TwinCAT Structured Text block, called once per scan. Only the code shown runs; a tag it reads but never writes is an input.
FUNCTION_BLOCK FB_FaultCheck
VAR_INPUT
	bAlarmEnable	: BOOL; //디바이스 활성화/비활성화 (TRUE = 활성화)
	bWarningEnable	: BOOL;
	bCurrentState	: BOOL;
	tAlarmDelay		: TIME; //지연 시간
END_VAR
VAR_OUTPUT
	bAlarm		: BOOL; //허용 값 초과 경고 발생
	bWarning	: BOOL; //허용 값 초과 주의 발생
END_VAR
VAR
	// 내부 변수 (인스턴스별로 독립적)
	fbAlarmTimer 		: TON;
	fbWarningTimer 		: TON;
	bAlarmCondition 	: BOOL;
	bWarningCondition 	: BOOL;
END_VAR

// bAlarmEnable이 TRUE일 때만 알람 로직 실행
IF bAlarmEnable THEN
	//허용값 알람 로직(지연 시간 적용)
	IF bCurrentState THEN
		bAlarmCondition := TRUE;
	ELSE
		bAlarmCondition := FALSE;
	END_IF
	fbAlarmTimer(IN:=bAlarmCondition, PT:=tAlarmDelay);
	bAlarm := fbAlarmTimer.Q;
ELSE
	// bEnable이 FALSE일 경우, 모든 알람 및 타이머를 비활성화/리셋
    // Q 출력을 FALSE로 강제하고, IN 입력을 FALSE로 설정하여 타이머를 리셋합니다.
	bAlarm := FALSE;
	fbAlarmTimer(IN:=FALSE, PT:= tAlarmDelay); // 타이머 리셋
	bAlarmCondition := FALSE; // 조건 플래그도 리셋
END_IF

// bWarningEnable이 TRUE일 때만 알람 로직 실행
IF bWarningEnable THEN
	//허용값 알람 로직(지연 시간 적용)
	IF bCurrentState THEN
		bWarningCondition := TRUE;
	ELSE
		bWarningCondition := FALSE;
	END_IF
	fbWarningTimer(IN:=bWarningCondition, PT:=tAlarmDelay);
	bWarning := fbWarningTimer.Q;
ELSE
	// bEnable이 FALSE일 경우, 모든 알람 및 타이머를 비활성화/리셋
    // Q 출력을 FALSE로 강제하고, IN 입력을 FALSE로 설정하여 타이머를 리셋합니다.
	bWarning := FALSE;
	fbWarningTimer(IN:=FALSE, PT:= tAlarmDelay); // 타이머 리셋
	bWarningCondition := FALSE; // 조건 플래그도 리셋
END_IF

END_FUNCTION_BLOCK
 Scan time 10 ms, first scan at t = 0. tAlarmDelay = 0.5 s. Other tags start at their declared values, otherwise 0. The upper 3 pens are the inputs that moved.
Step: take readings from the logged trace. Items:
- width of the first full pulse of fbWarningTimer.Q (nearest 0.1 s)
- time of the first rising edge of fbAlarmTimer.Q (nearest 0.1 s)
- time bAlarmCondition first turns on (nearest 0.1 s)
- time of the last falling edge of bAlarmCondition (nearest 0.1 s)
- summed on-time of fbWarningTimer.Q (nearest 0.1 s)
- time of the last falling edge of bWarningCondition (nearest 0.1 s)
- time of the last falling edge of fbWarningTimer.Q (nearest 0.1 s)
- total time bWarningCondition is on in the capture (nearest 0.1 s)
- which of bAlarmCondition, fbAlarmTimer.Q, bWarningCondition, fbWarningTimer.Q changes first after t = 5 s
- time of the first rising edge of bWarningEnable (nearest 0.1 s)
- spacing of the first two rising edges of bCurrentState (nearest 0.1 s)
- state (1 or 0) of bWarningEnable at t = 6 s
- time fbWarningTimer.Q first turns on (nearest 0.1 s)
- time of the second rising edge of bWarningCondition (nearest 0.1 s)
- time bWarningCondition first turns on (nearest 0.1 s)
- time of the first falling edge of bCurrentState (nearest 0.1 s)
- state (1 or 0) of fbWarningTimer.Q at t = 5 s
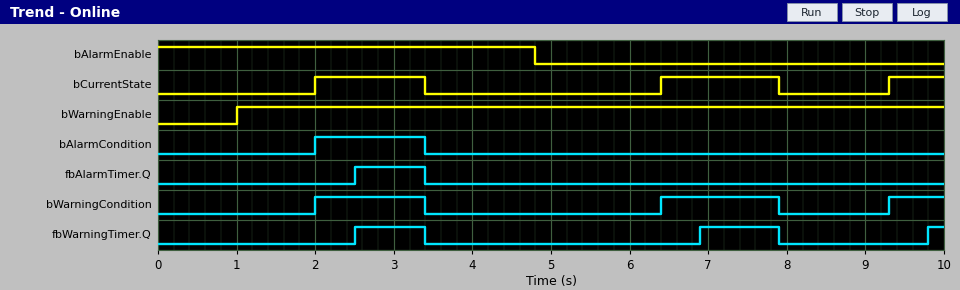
0.9 s
2.5 s
2.0 s
3.4 s
2.1 s
7.9 s
7.9 s
3.6 s
bWarningCondition
1.0 s
4.4 s
1
2.5 s
6.4 s
2.0 s
3.4 s
0
